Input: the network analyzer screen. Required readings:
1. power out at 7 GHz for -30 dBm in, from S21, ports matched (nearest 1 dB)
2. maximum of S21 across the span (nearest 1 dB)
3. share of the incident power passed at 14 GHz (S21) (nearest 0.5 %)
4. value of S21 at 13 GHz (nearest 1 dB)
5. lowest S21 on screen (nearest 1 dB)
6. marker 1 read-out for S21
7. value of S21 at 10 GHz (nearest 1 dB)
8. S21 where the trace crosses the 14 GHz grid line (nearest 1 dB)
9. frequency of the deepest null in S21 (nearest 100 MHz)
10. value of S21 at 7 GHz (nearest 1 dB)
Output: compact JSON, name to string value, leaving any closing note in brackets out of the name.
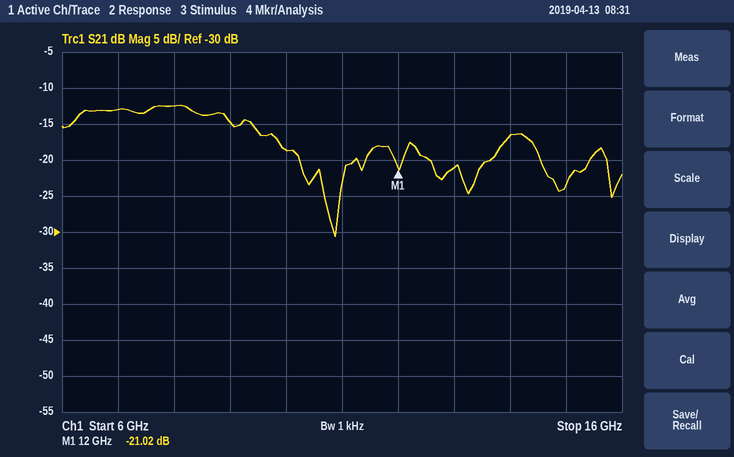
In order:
{"power out at 7 GHz for -30 dBm in, from S21, ports matched": "-43 dBm", "maximum of S21 across the span": "-12 dB", "share of the incident power passed at 14 GHz (S21)": "2.0 %", "value of S21 at 13 GHz": "-21 dB", "lowest S21 on screen": "-31 dB", "marker 1 read-out for S21": "-21.02 dB", "value of S21 at 10 GHz": "-19 dB", "S21 where the trace crosses the 14 GHz grid line": "-17 dB", "frequency of the deepest null in S21": "10.9 GHz", "value of S21 at 7 GHz": "-13 dB"}
